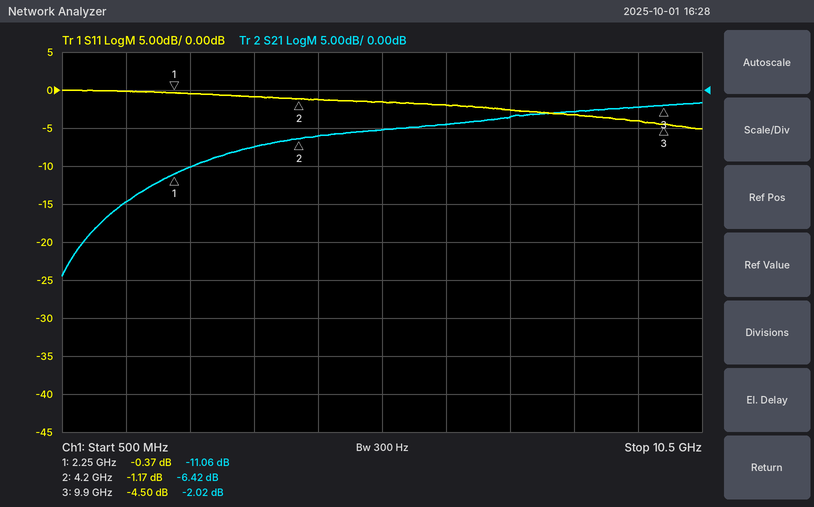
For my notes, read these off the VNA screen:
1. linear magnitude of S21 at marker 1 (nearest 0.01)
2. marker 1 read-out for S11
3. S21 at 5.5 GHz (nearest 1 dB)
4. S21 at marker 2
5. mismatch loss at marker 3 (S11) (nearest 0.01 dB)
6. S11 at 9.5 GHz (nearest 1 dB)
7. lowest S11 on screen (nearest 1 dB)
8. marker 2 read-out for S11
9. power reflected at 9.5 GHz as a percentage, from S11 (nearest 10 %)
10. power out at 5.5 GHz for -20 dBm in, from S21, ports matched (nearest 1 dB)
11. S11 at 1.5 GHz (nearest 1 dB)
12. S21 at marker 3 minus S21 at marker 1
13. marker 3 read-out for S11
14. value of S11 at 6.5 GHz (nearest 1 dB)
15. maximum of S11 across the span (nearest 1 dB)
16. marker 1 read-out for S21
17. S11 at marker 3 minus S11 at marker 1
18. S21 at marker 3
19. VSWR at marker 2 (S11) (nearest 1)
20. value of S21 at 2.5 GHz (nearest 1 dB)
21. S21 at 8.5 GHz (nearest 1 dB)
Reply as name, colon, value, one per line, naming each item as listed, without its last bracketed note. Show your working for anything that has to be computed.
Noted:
linear magnitude of S21 at marker 1: 10^(-11.06/20) ≈ 0.28
marker 1 read-out for S11: -0.37 dB
S21 at 5.5 GHz: -5 dB
S21 at marker 2: -6.42 dB
mismatch loss at marker 3 (S11): −10 log10(1 − 10^(-4.5/10)) ≈ 1.90 dB
S11 at 9.5 GHz: -4 dB
lowest S11 on screen: -5 dB
marker 2 read-out for S11: -1.17 dB
power reflected at 9.5 GHz as a percentage, from S11: 10^(-4/10) ≈ 40 %
power out at 5.5 GHz for -20 dBm in, from S21, ports matched: -20 dBm + (-5 dB) = -25 dBm
S11 at 1.5 GHz: 0 dB
S21 at marker 3 minus S21 at marker 1: -2.02 − (-11.06) = 9.04 dB
marker 3 read-out for S11: -4.50 dB
value of S11 at 6.5 GHz: -2 dB
maximum of S11 across the span: 0 dB
marker 1 read-out for S21: -11.06 dB
S11 at marker 3 minus S11 at marker 1: -4.5 − (-0.37) = -4.13 dB
S21 at marker 3: -2.02 dB
VSWR at marker 2 (S11): (1 + 0.8740)/(1 − 0.8740) ≈ 15
value of S21 at 2.5 GHz: -10 dB
S21 at 8.5 GHz: -3 dB
